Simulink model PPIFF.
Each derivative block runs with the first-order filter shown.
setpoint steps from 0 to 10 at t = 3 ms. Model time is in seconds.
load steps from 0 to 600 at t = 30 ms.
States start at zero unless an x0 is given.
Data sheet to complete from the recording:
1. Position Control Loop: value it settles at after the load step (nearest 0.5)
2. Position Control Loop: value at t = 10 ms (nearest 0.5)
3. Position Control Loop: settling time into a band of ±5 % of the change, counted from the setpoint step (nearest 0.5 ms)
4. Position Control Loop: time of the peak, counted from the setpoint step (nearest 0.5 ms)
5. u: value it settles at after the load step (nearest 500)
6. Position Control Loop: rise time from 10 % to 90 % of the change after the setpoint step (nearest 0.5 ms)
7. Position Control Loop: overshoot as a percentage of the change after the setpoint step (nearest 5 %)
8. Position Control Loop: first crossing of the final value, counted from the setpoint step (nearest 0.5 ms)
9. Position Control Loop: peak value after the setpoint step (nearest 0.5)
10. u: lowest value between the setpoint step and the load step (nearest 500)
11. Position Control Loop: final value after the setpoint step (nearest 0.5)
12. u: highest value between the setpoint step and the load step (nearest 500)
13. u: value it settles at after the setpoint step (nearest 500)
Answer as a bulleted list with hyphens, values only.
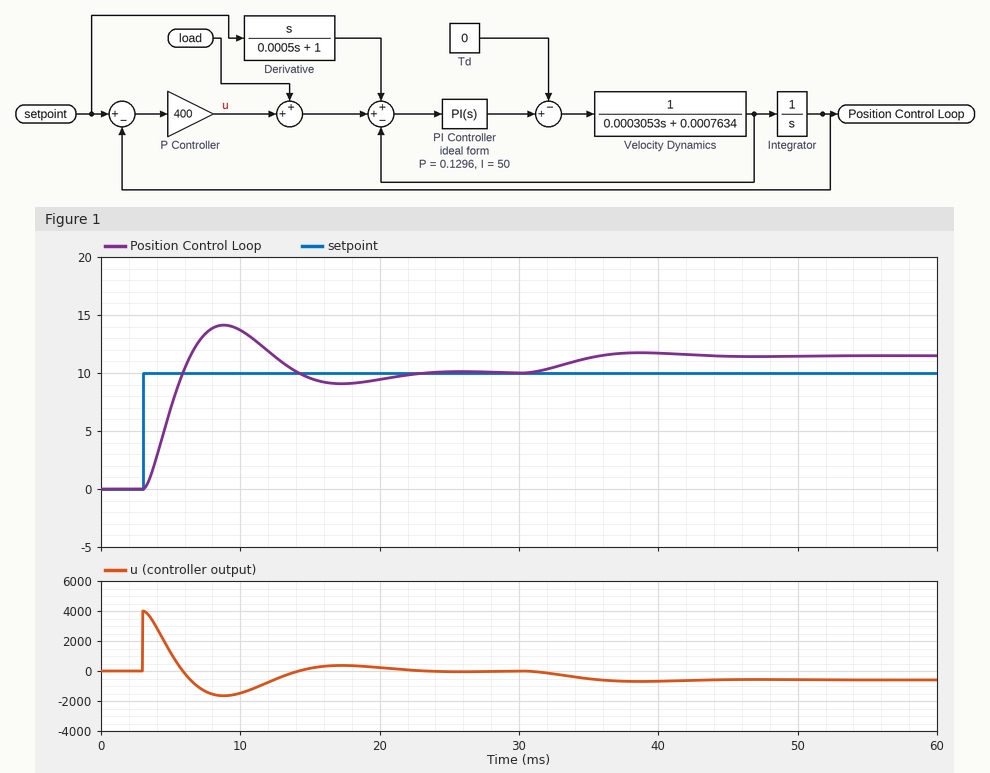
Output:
- 11.5
- 13.5
- 17.5 ms
- 6.0 ms
- -500
- 2.0 ms
- 40 %
- 3.0 ms
- 14.0
- -1500
- 10.0
- 4000
- 0
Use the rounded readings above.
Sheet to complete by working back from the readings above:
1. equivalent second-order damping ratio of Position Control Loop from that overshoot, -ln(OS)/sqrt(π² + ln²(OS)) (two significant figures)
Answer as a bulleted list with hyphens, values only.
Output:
- 0.28
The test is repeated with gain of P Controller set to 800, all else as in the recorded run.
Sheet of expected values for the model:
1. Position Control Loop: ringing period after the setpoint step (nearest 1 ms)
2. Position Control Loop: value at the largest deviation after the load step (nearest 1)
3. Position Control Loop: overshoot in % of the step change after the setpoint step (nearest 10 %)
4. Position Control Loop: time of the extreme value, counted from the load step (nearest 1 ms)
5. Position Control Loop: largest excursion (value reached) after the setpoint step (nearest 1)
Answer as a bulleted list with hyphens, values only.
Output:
- 11 ms
- 11
- 50 %
- 6 ms
- 15
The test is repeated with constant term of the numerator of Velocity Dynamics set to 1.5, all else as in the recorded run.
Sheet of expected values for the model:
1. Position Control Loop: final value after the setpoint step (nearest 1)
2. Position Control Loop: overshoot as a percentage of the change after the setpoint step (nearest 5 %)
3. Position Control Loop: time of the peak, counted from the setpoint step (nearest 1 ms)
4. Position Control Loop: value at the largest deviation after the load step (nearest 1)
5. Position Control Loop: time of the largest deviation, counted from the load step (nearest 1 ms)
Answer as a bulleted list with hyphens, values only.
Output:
- 10
- 35 %
- 5 ms
- 12
- 8 ms
